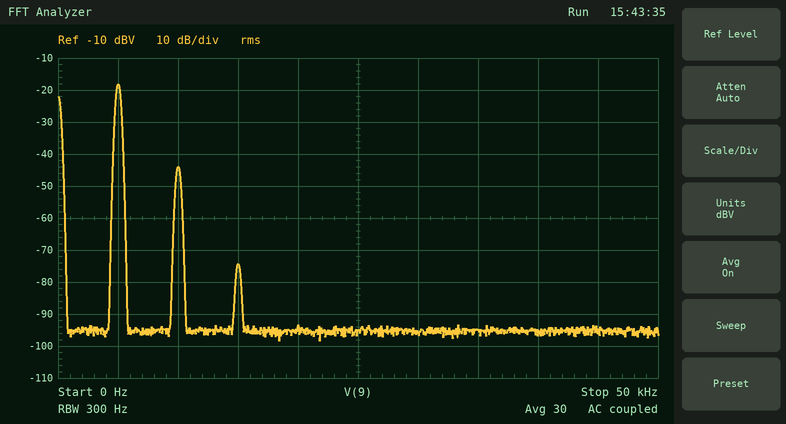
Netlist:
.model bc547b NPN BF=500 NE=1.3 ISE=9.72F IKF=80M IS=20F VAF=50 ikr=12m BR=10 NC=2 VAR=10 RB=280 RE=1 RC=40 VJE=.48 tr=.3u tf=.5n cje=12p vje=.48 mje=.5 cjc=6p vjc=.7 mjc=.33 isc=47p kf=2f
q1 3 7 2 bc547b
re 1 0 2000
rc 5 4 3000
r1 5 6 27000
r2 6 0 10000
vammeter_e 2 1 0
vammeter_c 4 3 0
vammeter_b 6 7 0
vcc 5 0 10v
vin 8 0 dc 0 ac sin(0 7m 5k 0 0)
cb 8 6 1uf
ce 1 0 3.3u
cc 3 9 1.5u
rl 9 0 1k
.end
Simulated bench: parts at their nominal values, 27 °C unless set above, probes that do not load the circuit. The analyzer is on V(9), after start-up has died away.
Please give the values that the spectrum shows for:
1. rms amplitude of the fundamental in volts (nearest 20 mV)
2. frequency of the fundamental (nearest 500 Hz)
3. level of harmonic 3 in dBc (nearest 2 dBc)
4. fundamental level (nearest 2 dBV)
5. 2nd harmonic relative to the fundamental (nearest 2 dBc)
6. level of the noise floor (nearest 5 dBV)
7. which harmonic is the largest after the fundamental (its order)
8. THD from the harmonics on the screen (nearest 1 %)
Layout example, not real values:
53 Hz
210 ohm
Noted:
120 mV
5.0 kHz
-56 dBc
-18 dBV
-26 dBc
-95 dBV
2
5 %
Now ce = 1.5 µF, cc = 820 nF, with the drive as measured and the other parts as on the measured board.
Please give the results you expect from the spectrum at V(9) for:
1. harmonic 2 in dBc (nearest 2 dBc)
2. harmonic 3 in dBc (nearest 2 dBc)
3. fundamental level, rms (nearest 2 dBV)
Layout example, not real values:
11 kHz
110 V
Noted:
-28 dBc
-58 dBc
-20 dBV
